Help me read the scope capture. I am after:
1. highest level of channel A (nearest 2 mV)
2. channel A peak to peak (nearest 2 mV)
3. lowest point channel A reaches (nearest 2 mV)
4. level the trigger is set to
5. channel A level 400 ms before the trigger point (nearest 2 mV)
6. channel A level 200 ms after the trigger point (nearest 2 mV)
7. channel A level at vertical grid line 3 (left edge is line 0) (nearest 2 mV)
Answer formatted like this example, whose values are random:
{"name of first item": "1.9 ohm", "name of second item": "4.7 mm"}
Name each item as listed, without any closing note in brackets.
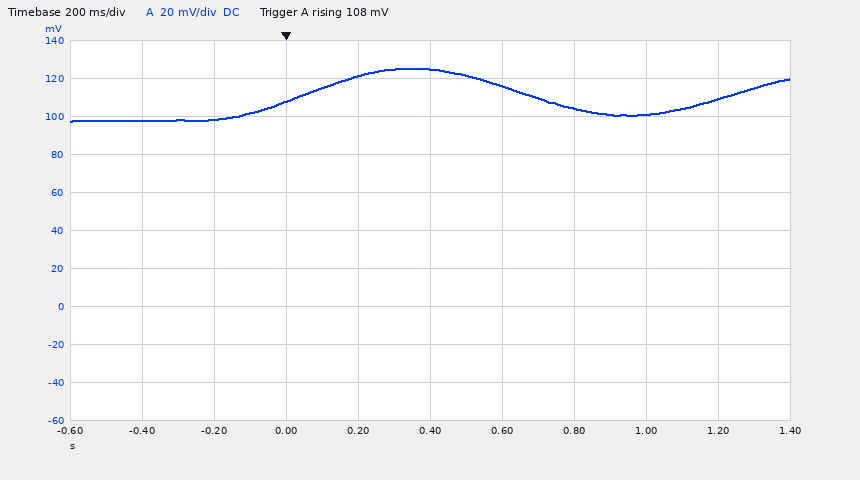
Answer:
{"highest level of channel A": "126 mV", "channel A peak to peak": "28 mV", "lowest point channel A reaches": "98 mV", "level the trigger is set to": "108 mV", "channel A level 400 ms before the trigger point": "98 mV", "channel A level 200 ms after the trigger point": "122 mV", "channel A level at vertical grid line 3 (left edge is line 0)": "108 mV"}
